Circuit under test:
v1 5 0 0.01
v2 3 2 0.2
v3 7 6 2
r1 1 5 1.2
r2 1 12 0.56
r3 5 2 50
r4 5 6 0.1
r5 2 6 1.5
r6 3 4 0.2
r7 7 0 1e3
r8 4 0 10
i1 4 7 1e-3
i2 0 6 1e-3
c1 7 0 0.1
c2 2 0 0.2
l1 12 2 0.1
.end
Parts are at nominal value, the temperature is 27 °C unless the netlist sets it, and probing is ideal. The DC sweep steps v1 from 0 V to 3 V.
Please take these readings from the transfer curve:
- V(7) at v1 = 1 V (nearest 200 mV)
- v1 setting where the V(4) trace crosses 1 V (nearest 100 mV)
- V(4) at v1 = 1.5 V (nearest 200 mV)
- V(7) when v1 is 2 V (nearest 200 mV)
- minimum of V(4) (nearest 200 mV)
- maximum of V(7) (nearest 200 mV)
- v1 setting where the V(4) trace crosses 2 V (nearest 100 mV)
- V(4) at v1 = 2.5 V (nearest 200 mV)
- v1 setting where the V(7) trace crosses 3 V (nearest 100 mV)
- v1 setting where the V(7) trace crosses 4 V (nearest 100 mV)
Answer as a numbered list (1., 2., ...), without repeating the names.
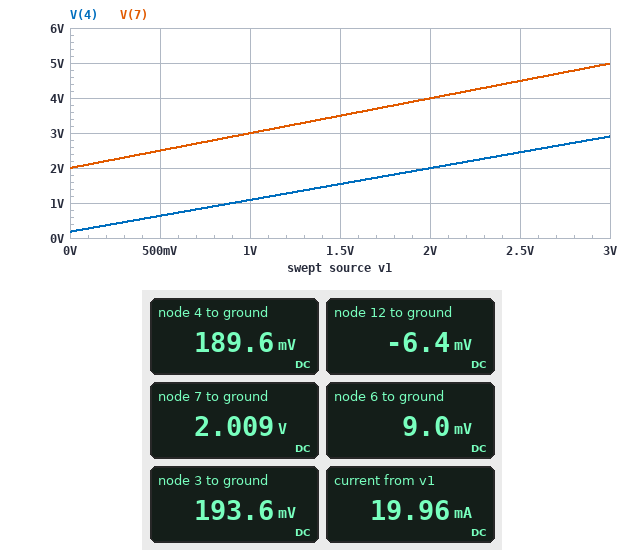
1. 3.0 V
2. 900 mV
3. 1.6 V
4. 4.0 V
5. 200 mV
6. 5.0 V
7. 2.0 V
8. 2.4 V
9. 1.0 V
10. 2.0 V
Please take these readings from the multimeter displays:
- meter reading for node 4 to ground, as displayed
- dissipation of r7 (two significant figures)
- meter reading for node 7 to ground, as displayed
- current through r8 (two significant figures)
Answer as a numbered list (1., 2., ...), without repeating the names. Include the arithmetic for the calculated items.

1. 189.6 mV
2. (2.009 V)^2 / 1 kΩ = 4.0 mW
3. 2.009 V
4. (189.6 mV) / 10 Ω = 19 mA
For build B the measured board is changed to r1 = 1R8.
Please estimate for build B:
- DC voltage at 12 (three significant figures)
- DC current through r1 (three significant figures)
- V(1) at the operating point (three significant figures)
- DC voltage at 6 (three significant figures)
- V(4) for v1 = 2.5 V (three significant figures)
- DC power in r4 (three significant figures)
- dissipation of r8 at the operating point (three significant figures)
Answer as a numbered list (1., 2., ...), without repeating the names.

1. -8.49 mV
2. 7.83 mA
3. -4.10 mV
4. 8.84 mV
5. 2.42 V
6. 13.4 µW
7. 3.52 mW
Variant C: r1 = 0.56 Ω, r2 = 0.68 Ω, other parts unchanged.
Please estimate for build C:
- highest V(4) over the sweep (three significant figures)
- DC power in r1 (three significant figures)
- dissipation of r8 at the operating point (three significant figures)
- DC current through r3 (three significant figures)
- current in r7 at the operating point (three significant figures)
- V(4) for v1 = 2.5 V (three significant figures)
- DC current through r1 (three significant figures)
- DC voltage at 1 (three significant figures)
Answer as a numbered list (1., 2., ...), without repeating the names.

1. 2.94 V
2. 70.6 µW
3. 3.69 mW
4. 278 µA
5. 2.01 mA
6. 2.48 V
7. 11.2 mA
8. 3.71 mV
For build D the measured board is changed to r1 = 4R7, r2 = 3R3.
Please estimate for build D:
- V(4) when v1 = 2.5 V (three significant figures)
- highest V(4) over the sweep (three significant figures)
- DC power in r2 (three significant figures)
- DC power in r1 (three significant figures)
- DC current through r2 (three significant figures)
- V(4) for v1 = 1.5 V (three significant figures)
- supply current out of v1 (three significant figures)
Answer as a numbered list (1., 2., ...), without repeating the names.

1. 2.35 V
2. 2.78 V
3. 31.8 µW
4. 45.3 µW
5. 3.11 mA
6. 1.48 V
7. 19.1 mA
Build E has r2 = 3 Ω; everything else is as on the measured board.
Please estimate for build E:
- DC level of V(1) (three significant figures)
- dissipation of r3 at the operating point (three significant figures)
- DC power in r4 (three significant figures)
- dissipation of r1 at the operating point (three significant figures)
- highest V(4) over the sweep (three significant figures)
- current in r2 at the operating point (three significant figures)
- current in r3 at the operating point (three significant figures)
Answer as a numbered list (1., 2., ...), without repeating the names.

1. 3.72 mV
2. 9.67 µW
3. 18.9 µW
4. 32.9 µW
5. 2.82 V
6. 5.23 mA
7. 440 µA
